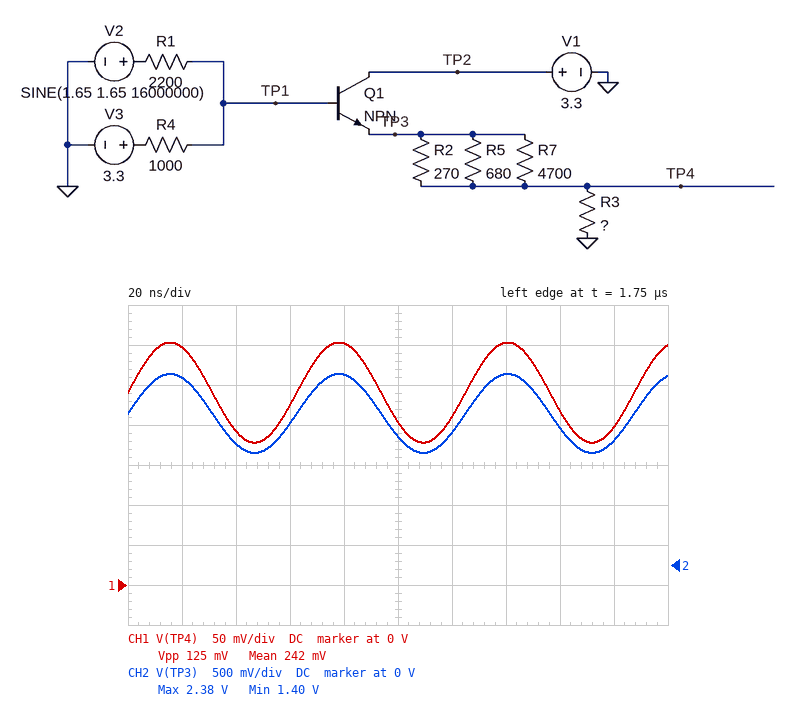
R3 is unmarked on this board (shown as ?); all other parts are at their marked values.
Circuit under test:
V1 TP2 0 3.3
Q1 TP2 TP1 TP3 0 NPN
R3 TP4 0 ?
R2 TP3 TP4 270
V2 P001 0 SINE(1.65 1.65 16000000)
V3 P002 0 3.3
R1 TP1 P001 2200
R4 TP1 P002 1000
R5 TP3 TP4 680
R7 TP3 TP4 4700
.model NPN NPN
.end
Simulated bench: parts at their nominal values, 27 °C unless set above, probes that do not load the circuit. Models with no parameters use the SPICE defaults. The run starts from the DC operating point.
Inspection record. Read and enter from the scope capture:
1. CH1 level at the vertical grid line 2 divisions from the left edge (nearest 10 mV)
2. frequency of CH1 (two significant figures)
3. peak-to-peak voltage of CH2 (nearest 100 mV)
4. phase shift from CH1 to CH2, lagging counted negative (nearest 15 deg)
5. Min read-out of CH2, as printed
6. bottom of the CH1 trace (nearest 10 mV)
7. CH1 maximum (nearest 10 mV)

190 mV
16 MHz
1.0 V
0 deg
1.40 V
180 mV
300 mV
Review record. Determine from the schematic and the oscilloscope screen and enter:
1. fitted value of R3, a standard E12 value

27 Ω
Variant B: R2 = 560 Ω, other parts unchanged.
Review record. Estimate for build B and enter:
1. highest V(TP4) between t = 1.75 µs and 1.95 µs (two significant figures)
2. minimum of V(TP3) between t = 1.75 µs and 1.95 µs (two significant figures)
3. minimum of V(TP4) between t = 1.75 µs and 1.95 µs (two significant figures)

210 mV
1.4 V
120 mV
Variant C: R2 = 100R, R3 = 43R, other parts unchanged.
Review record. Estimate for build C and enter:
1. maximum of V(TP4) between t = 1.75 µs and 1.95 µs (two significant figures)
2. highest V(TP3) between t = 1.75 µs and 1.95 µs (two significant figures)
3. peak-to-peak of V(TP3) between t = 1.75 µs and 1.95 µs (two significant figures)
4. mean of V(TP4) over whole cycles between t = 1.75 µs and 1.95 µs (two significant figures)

780 mV
2.3 V
970 mV
620 mV
